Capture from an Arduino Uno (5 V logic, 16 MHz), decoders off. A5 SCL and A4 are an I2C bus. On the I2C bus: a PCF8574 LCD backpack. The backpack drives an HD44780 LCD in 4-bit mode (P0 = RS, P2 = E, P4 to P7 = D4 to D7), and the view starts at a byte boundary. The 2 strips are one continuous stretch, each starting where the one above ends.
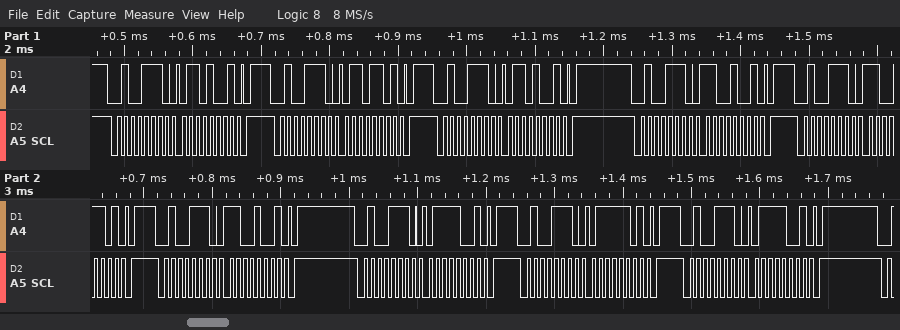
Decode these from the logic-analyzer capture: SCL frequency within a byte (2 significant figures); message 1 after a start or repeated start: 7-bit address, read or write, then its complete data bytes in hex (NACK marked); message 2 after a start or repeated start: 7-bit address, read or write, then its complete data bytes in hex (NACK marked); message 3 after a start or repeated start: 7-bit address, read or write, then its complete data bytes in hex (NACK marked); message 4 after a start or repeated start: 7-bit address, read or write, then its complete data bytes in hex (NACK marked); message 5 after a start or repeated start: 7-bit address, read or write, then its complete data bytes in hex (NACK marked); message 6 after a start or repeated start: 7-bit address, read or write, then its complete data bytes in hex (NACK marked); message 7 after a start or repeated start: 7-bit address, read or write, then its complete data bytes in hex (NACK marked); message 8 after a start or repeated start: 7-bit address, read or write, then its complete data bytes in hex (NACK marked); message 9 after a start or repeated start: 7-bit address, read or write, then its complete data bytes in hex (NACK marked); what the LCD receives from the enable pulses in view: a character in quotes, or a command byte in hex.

100 kHz
0x27 write: 69
0x27 write: 6D
0x27 write: 69
0x27 write: C9
0x27 write: CD
0x27 write: C9
0x27 write: 79
0x27 write: 7D
0x27 write: 79
'l'
